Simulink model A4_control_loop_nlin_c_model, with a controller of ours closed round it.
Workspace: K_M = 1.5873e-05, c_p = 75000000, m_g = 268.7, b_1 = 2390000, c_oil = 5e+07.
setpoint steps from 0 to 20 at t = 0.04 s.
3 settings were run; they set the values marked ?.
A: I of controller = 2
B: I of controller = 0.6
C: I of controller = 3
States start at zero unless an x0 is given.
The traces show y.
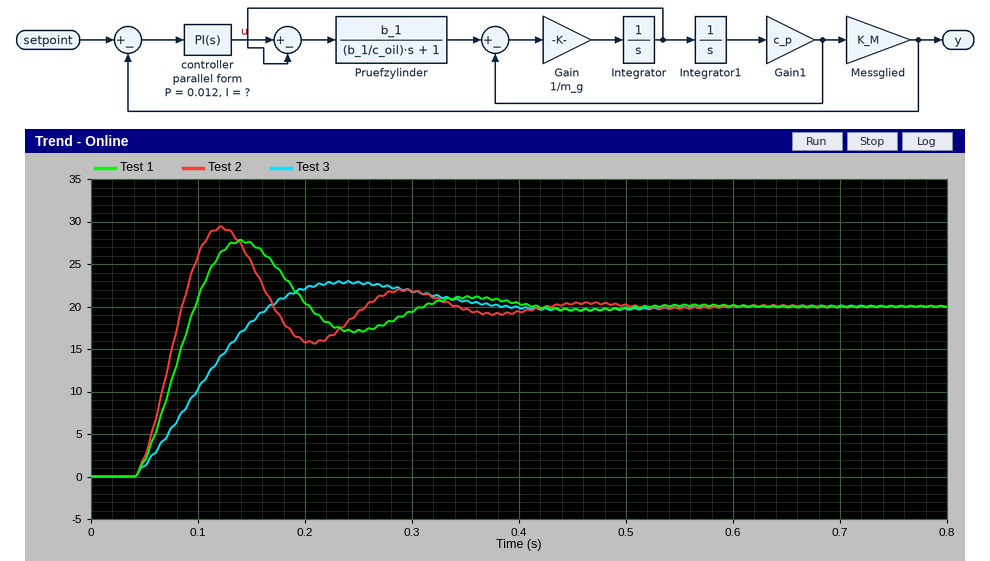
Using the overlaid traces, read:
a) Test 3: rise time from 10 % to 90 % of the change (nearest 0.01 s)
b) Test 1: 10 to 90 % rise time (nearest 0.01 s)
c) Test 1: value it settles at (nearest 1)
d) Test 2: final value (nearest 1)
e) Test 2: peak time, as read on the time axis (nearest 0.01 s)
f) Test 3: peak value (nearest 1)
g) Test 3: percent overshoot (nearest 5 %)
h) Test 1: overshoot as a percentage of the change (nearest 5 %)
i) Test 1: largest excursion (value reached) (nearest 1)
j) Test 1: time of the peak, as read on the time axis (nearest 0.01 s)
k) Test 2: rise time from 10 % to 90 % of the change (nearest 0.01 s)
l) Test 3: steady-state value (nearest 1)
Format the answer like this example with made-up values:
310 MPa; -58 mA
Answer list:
0.09 s; 0.04 s; 20; 20; 0.12 s; 23; 15 %; 40 %; 28; 0.14 s; 0.03 s; 20
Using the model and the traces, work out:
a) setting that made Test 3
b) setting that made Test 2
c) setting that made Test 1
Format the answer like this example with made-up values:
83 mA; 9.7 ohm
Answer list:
B; C; A
